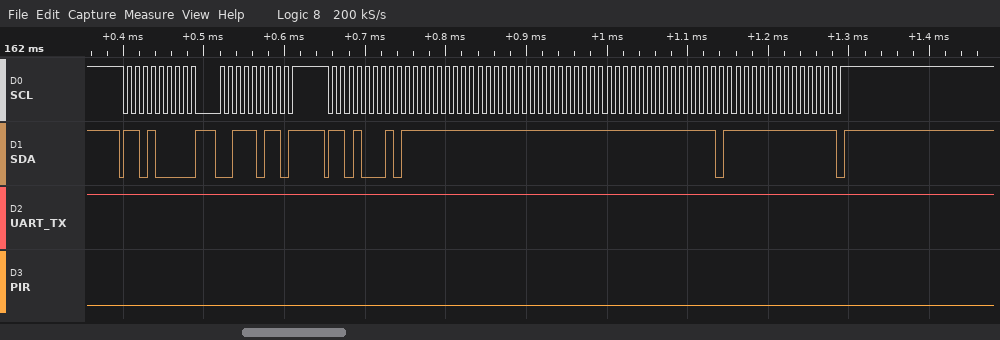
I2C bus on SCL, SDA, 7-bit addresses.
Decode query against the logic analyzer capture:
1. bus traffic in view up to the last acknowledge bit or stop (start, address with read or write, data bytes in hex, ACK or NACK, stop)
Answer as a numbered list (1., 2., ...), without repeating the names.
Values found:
1. start, address 68 write ACK, 3B ACK, repeated start, address 68 read ACK, FF NACK, FF NACK, FF NACK, FF NACK, EF NACK, FF NACK, stop
